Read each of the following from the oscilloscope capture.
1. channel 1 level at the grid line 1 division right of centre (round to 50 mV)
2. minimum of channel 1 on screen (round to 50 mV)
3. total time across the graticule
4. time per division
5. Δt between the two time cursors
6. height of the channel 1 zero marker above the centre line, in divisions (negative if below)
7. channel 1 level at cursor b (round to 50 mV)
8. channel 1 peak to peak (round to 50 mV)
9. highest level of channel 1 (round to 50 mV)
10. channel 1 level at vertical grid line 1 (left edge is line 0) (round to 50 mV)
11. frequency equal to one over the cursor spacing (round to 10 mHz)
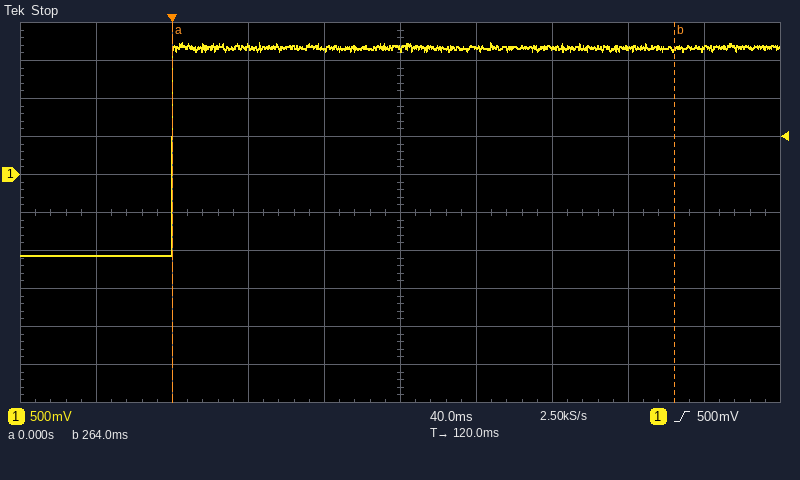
1.65 V
-1.05 V
400 ms
40 ms
264 ms
+1.0 div
1.65 V
2.80 V
1.75 V
-1.05 V
3.79 Hz
